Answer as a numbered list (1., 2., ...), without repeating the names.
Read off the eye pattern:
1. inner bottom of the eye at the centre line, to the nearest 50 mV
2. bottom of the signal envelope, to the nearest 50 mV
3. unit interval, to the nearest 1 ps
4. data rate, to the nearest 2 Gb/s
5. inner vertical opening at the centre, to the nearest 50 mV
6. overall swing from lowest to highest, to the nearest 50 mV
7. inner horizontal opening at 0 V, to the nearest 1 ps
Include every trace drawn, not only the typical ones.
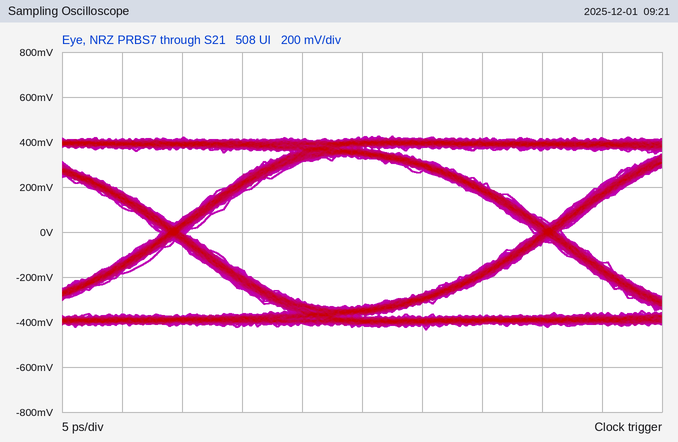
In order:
1. -350 mV
2. -450 mV
3. 31 ps
4. 32 Gb/s
5. 650 mV
6. 850 mV
7. 29 ps
